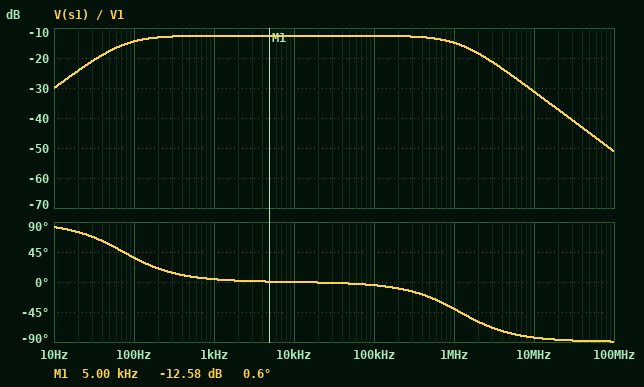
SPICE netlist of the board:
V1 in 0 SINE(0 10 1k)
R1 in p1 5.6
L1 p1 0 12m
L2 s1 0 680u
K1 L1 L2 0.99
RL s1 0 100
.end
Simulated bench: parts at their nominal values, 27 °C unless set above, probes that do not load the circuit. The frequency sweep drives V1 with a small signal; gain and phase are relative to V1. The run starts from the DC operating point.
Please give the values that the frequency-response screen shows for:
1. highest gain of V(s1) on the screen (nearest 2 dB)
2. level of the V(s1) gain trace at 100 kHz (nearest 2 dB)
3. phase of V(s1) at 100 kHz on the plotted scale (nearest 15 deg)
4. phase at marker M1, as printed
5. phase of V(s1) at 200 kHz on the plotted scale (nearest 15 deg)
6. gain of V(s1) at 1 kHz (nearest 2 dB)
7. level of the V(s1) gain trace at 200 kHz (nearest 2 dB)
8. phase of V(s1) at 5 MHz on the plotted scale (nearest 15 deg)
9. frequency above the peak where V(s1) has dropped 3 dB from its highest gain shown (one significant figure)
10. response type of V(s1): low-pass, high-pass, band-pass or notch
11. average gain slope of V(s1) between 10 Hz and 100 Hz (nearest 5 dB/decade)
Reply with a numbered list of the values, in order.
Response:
1. -12 dB
2. -12 dB
3. 0 deg
4. 0.6 deg
5. -15 deg
6. -12 dB
7. -12 dB
8. -75 deg
9. 1 MHz
10. band-pass
11. 15 dB/decade
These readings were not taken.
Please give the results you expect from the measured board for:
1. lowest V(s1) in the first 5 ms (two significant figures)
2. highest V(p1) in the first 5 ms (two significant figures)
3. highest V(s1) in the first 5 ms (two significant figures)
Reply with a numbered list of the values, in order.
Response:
1. -2.5 V
2. 9.8 V
3. 2.3 V
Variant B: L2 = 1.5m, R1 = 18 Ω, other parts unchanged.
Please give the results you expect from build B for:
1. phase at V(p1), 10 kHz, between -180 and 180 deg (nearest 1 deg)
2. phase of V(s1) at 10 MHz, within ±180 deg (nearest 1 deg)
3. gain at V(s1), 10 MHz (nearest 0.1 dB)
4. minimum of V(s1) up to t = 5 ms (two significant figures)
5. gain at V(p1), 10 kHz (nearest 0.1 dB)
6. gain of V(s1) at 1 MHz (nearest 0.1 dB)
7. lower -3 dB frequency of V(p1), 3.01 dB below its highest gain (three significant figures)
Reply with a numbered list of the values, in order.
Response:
1. 1 deg
2. -87 deg
3. -34.6 dB
4. -3.6 V
5. -0.2 dB
6. -15.7 dB
7. 244 Hz
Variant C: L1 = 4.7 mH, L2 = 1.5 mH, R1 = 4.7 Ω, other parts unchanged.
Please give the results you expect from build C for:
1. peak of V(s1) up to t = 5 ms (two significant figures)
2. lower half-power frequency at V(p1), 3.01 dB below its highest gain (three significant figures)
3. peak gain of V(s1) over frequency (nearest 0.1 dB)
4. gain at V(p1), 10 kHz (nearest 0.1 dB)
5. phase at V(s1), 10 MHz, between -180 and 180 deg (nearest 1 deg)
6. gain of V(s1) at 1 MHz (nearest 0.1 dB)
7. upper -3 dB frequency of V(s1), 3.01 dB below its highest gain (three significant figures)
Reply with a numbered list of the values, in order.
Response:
1. 5.4 V
2. 162 Hz
3. -5.2 dB
4. -0.1 dB
5. -87 deg
6. -11.6 dB
7. 541 kHz
